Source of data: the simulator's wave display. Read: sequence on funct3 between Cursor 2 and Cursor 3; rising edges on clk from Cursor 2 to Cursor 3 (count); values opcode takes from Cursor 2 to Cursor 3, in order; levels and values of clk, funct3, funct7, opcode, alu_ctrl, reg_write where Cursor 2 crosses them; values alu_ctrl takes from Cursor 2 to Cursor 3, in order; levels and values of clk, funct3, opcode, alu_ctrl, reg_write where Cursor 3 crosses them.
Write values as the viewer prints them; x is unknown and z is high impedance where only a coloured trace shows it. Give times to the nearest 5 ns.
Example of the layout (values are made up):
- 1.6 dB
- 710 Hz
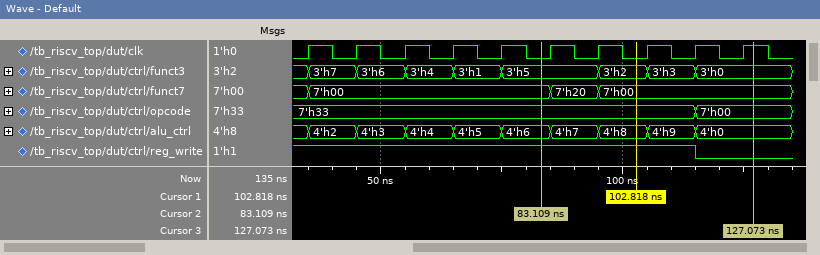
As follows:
- 3'h5, 3'h2, 3'h3, 3'h0
- 5
- 7'h33, 7'h00
- clk=0, funct3=3'h5, funct7=7'h00, opcode=7'h33, alu_ctrl=4'h6, reg_write=1
- 4'h6, 4'h7, 4'h8, 4'h9, 4'h0
- clk=1, funct3=3'h0, opcode=7'h00, alu_ctrl=4'h0, reg_write=0
